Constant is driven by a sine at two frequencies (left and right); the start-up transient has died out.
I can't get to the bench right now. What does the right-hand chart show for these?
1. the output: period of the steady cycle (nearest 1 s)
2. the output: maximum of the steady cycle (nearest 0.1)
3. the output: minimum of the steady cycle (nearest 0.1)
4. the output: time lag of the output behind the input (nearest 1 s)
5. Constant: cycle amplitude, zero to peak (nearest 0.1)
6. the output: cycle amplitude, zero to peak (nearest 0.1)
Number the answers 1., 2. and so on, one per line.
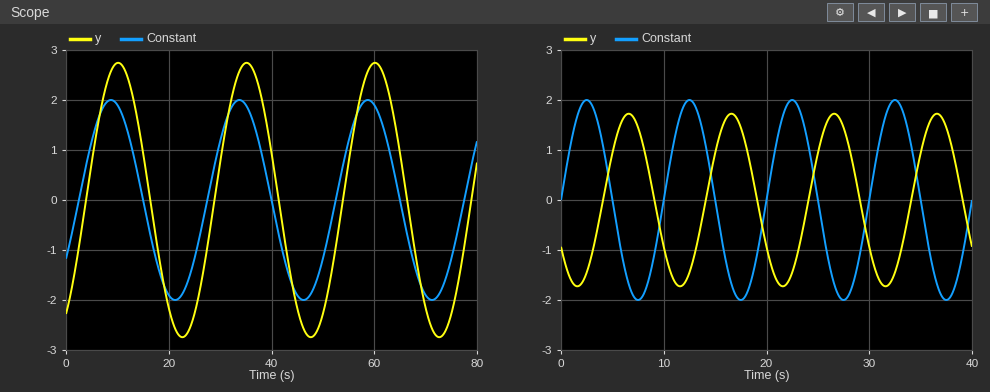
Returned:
1. 10 s
2. 1.7
3. -1.7
4. 4 s
5. 2.0
6. 1.7
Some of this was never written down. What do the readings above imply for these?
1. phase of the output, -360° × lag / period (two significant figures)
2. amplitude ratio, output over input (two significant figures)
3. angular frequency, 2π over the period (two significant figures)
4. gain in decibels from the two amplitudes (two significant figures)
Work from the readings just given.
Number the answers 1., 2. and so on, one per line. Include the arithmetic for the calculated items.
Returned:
1. -360 × 4 / 10 = -140°
2. 1.7 / 2 = 0.85
3. 2π / 10 = 0.63 rad/s
4. 20 log10(1.7 / 2) = -1.4 dB
